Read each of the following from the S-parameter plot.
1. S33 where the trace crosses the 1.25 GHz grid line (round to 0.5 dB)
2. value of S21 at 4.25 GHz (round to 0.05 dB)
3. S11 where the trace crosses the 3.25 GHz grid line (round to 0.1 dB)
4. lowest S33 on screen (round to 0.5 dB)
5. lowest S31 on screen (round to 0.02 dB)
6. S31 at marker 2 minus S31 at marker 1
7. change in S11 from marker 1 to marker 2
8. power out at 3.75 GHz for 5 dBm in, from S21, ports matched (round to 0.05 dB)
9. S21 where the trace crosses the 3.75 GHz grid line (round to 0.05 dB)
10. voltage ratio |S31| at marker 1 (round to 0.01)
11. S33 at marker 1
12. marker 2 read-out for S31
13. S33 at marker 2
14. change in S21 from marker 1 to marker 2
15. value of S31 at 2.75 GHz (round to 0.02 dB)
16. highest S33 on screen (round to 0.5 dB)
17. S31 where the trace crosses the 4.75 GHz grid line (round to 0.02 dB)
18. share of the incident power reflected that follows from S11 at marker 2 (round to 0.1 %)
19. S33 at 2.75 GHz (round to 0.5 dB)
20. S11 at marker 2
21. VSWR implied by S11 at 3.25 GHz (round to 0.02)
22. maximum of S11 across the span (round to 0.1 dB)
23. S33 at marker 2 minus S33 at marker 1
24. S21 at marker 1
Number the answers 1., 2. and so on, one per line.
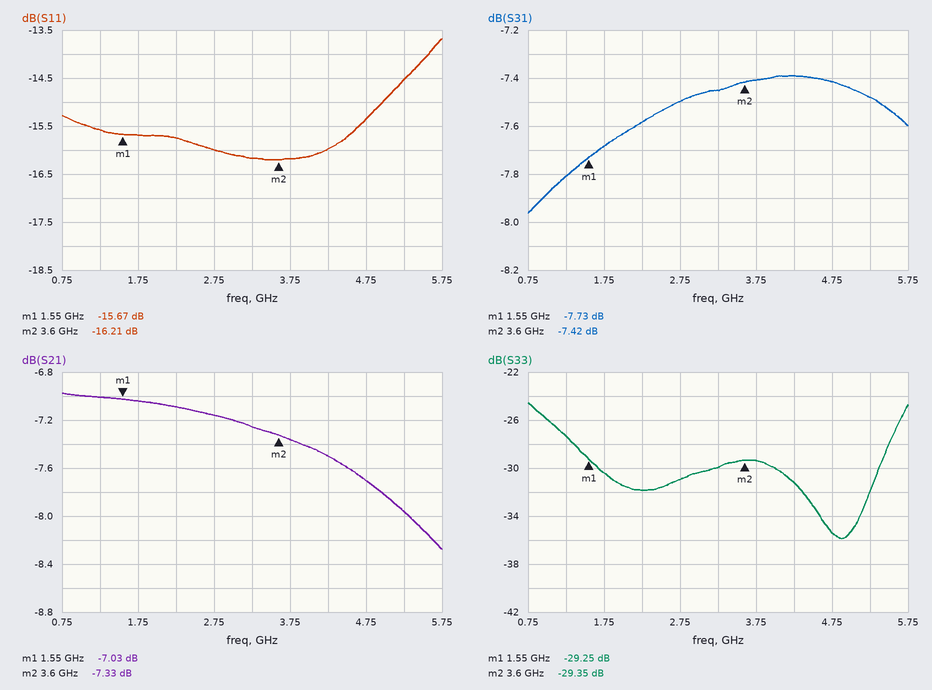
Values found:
1. -27.5 dB
2. -7.50 dB
3. -16.2 dB
4. -36.0 dB
5. -7.96 dB
6. 0.31 dB
7. -0.54 dB
8. -2.35 dBm
9. -7.35 dB
10. 0.41
11. -29.25 dB
12. -7.42 dB
13. -29.35 dB
14. -0.30 dB
15. -7.50 dB
16. -24.5 dB
17. -7.42 dB
18. 2.4 %
19. -31.0 dB
20. -16.21 dB
21. 1.36
22. -13.7 dB
23. -0.10 dB
24. -7.03 dB
